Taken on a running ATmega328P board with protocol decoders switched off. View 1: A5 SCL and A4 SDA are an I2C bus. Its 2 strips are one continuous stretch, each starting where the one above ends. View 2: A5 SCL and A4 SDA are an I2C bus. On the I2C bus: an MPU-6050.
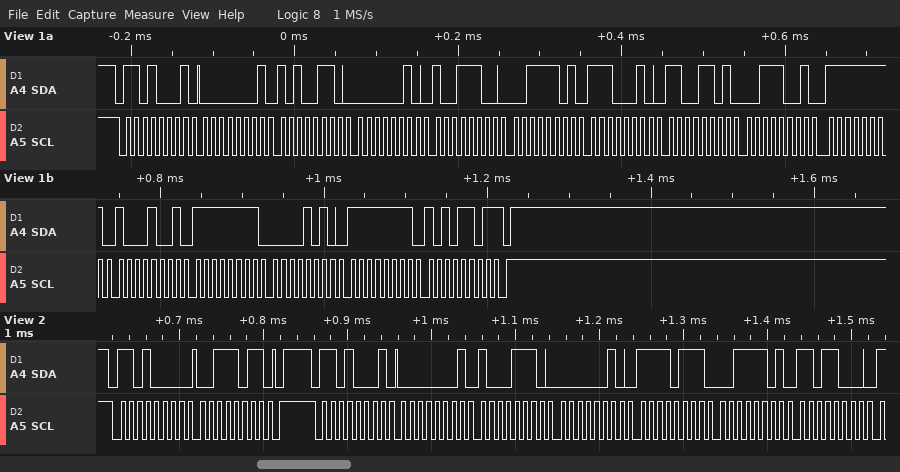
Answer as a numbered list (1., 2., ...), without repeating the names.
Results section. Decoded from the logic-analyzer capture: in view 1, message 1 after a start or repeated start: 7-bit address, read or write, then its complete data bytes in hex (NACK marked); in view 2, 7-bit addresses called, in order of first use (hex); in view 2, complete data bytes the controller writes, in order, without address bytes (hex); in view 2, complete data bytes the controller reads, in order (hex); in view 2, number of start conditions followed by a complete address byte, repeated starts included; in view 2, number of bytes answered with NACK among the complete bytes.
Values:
1. 0x68 read: 01 A6 02 9C 3D E2 CD 39 FF 89 FF 0A FF AD NACK
2. 0x68
3. 3B
4. 01 8E 02 F7 3D D8
5. 2
6. 0
